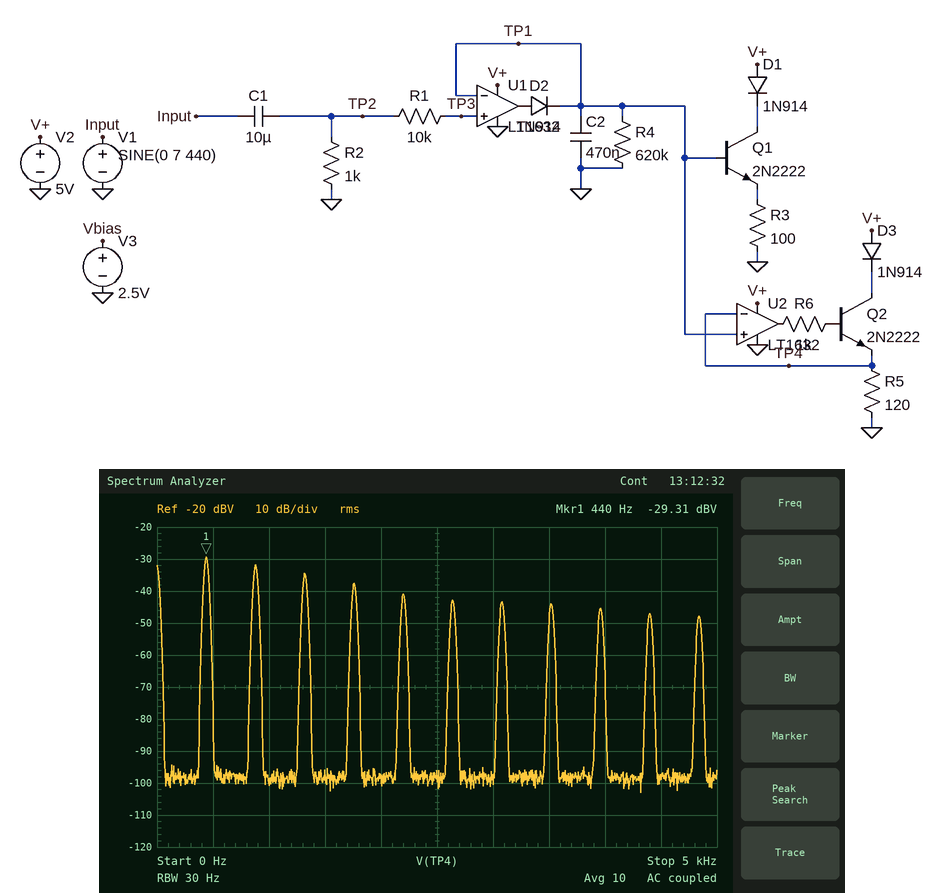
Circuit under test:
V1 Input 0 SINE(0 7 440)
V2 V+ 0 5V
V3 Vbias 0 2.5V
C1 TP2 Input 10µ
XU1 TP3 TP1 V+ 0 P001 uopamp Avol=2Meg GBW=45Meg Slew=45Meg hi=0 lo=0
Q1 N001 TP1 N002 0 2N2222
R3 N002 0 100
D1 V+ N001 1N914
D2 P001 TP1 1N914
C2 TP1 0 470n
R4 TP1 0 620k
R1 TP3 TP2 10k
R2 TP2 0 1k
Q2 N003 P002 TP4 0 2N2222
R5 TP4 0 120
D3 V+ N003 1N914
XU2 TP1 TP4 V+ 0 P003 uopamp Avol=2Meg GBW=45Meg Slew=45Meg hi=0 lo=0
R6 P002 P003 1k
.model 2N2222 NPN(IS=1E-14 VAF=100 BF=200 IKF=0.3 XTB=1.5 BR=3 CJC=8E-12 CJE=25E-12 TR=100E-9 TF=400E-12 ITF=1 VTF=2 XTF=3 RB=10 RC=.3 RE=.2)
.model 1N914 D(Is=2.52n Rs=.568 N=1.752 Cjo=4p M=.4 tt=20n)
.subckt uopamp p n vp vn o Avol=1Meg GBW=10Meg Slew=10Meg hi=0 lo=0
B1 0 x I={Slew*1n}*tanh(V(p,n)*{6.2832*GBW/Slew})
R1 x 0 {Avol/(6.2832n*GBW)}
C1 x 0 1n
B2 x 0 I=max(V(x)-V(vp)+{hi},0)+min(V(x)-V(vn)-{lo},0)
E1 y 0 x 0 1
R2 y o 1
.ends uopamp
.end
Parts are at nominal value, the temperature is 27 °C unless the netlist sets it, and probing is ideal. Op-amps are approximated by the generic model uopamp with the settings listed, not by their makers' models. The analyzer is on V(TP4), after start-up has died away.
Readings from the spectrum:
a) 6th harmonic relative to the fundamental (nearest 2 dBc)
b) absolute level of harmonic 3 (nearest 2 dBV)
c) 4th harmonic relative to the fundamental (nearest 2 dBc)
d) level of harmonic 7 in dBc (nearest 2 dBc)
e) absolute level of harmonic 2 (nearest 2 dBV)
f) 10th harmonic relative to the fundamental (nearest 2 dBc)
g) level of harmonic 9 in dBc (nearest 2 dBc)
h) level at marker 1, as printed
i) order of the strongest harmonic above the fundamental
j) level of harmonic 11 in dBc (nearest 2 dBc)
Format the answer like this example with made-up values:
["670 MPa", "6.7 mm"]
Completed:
["-14 dBc", "-34 dBV", "-8 dBc", "-14 dBc", "-32 dBV", "-18 dBc", "-16 dBc", "-29.31 dBV", "2", "-18 dBc"]
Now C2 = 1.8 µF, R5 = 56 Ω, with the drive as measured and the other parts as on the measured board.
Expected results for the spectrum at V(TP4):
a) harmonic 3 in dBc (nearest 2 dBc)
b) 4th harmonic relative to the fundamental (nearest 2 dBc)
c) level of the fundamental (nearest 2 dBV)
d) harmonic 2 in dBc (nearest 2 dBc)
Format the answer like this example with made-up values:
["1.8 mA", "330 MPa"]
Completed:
["-10 dBc", "-12 dBc", "-90 dBV", "-6 dBc"]
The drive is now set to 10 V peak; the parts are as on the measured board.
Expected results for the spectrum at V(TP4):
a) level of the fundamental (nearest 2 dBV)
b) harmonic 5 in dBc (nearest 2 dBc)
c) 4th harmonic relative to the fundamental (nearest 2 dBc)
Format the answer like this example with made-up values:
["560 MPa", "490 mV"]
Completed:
["-34 dBV", "-8 dBc", "-6 dBc"]
